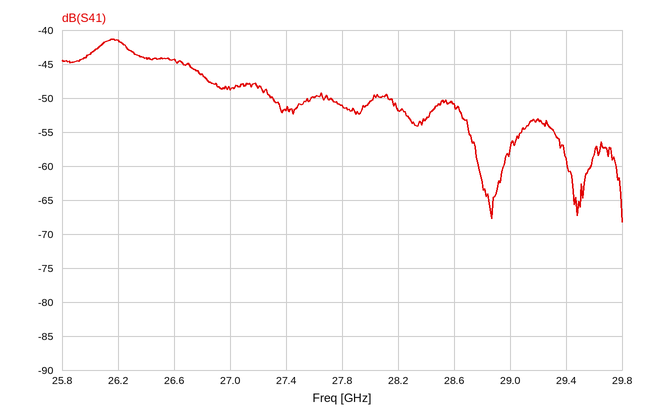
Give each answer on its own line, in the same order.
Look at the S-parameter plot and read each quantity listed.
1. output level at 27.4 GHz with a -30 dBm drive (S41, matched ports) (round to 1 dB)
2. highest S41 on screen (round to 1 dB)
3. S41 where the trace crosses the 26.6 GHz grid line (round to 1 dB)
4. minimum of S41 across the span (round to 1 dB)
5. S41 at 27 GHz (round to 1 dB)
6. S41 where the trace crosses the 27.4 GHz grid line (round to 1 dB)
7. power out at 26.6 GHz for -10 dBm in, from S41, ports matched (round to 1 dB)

-82 dBm
-41 dB
-44 dB
-68 dB
-49 dB
-52 dB
-54 dBm
